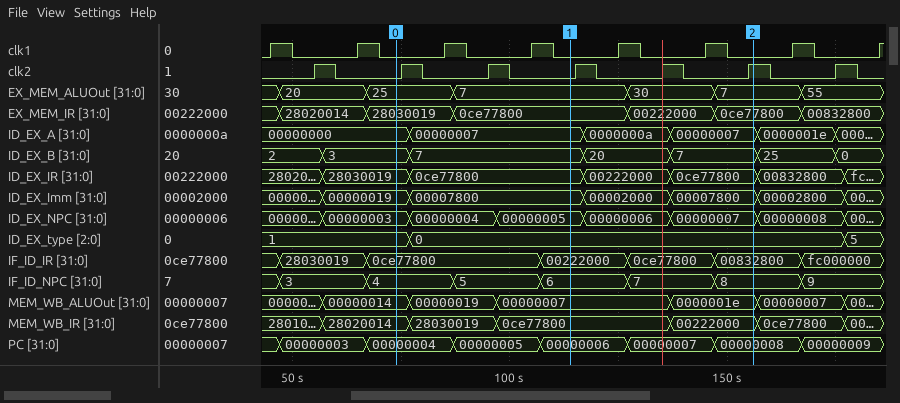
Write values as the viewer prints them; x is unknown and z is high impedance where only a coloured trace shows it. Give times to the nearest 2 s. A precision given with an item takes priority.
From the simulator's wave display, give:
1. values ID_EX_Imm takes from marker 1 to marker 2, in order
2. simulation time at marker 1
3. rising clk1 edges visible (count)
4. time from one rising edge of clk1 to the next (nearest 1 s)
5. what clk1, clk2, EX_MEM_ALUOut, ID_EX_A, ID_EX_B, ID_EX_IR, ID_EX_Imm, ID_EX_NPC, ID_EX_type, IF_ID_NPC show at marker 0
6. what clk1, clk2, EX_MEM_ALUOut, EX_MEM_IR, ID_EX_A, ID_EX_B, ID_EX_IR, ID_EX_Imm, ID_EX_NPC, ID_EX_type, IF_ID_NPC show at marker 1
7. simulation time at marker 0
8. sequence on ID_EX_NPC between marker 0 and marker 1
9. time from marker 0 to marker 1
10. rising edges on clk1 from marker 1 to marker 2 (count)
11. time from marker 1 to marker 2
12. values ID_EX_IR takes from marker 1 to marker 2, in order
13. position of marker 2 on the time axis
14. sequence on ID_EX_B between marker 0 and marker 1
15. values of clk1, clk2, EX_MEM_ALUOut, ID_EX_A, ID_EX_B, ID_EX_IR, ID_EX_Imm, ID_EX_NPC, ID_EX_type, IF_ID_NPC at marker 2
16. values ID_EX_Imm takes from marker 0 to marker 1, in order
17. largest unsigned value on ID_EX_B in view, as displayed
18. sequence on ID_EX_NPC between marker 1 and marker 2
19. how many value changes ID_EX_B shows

00007800, 00002000, 00007800
114 s
8
20 s
clk1=0, clk2=0, EX_MEM_ALUOut=25, ID_EX_A=00000000, ID_EX_B=3, ID_EX_IR=28030019, ID_EX_Imm=00000019, ID_EX_NPC=00000003, ID_EX_type=1, IF_ID_NPC=4
clk1=0, clk2=0, EX_MEM_ALUOut=7, EX_MEM_IR=0ce77800, ID_EX_A=00000007, ID_EX_B=7, ID_EX_IR=0ce77800, ID_EX_Imm=00007800, ID_EX_NPC=00000005, ID_EX_type=0, IF_ID_NPC=6
74 s
00000003, 00000004, 00000005
40 s
2
42 s
0ce77800, 00222000, 0ce77800
156 s
3, 7
clk1=0, clk2=1, EX_MEM_ALUOut=7, ID_EX_A=00000007, ID_EX_B=7, ID_EX_IR=0ce77800, ID_EX_Imm=00007800, ID_EX_NPC=00000007, ID_EX_type=0, IF_ID_NPC=8
00000019, 00007800
25
00000005, 00000006, 00000007
6
